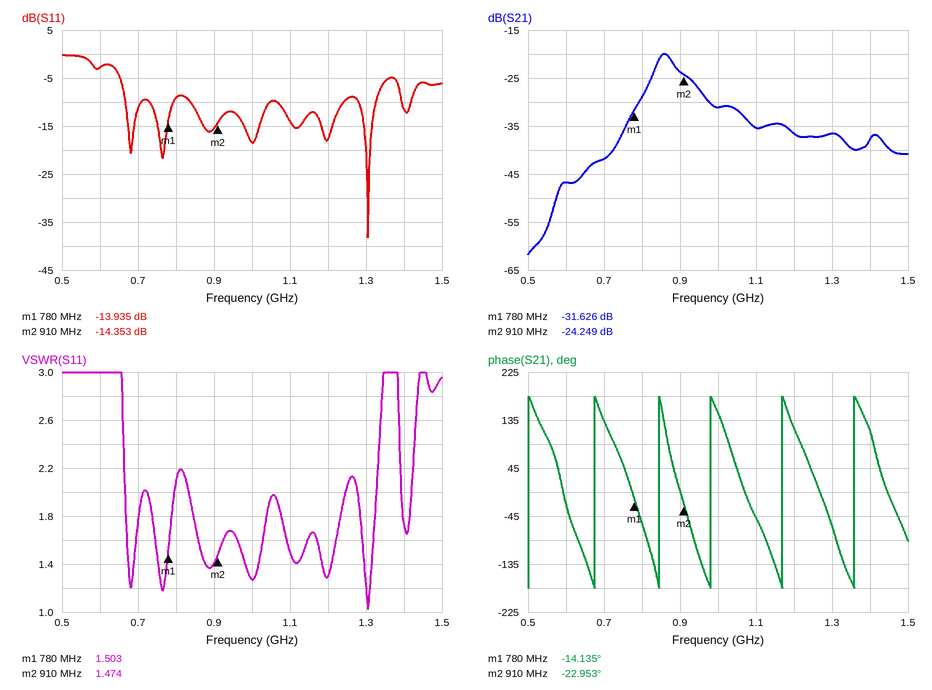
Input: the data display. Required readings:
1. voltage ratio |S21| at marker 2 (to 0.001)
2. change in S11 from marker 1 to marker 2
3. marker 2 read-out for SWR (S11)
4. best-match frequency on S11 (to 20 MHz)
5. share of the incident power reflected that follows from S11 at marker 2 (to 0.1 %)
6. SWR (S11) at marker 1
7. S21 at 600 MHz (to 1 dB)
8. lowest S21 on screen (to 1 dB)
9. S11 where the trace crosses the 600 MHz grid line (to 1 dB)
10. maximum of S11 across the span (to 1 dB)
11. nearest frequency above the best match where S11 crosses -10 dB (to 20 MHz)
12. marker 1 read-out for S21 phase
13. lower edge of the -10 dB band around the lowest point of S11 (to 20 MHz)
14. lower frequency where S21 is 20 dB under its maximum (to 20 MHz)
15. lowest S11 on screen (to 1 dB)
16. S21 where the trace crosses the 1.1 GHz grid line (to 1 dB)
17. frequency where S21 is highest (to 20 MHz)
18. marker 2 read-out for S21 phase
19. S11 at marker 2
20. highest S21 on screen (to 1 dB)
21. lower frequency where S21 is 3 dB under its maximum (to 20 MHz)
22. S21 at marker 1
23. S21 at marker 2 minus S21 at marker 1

0.061
-0.418 dB
1.474
1.30 GHz
3.7 %
1.503
-47 dB
-62 dB
-3 dB
0 dB
1.32 GHz
-14.135°
1.28 GHz
720 MHz
-38 dB
-35 dB
860 MHz
-22.953°
-14.353 dB
-20 dB
840 MHz
-31.626 dB
7.377 dB
